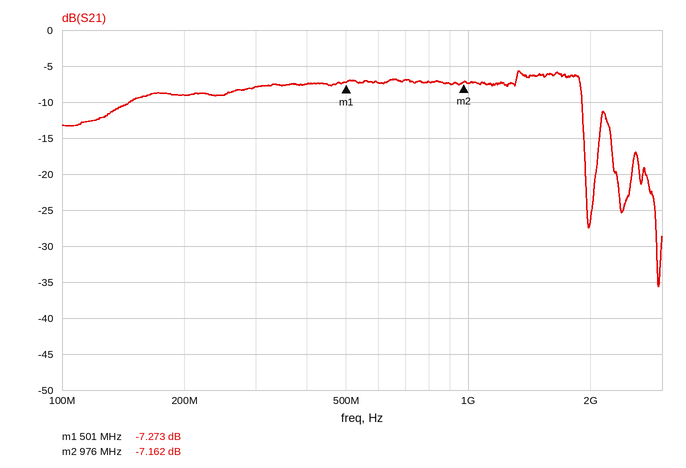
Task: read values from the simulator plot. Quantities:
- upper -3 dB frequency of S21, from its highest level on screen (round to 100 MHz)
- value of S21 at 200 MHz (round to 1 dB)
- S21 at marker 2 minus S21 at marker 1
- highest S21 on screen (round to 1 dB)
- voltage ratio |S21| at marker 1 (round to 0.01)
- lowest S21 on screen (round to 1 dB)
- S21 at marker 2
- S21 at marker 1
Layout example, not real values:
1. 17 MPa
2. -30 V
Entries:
1. 1.9 GHz
2. -9 dB
3. 0.111 dB
4. -6 dB
5. 0.43
6. -36 dB
7. -7.162 dB
8. -7.273 dB
